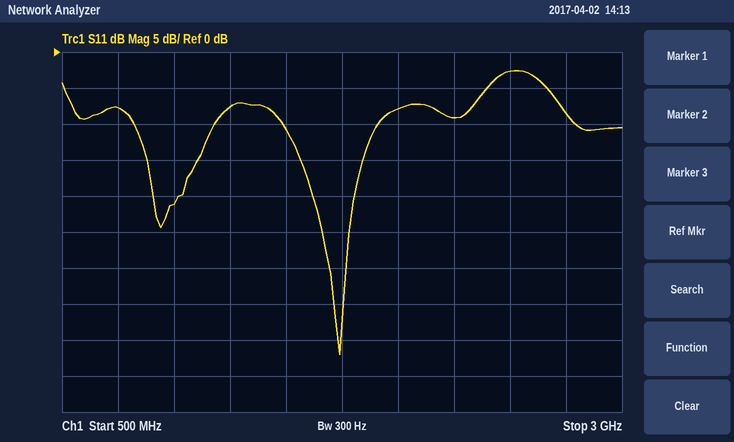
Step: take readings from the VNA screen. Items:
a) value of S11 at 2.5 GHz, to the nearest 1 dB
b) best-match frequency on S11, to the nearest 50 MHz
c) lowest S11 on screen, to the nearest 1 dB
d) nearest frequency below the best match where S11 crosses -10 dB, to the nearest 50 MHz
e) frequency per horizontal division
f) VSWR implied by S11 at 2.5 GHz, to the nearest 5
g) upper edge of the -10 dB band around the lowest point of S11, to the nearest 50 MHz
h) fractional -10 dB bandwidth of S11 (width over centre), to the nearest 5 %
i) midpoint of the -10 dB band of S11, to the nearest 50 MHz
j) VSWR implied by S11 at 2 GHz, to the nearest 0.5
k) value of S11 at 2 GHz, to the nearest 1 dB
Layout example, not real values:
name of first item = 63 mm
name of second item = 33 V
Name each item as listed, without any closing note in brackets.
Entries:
value of S11 at 2.5 GHz, to the nearest 1 dB = -3 dB
best-match frequency on S11, to the nearest 50 MHz = 1.75 GHz
lowest S11 on screen, to the nearest 1 dB = -42 dB
nearest frequency below the best match where S11 crosses -10 dB, to the nearest 50 MHz = 1.50 GHz
frequency per horizontal division = 250 MHz
VSWR implied by S11 at 2.5 GHz, to the nearest 5 = 5
upper edge of the -10 dB band around the lowest point of S11, to the nearest 50 MHz = 1.90 GHz
fractional -10 dB bandwidth of S11 (width over centre), to the nearest 5 % = 25 %
midpoint of the -10 dB band of S11, to the nearest 50 MHz = 1.70 GHz
VSWR implied by S11 at 2 GHz, to the nearest 0.5 = 2.5
value of S11 at 2 GHz, to the nearest 1 dB = -8 dB
